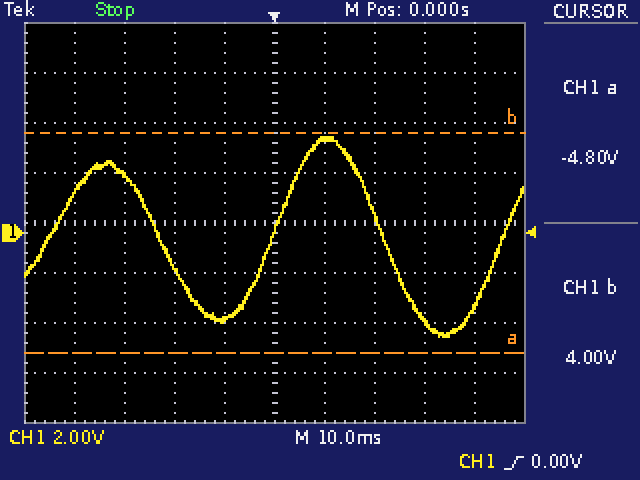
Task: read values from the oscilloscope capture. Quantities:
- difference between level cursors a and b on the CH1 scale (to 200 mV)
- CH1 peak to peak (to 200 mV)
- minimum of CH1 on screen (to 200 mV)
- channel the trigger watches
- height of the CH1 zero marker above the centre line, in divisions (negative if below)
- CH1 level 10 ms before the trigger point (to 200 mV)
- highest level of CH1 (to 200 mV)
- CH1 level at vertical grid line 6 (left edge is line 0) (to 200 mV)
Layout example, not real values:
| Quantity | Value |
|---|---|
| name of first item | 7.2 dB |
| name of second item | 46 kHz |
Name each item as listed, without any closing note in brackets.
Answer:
| Quantity | Value |
|---|---|
| difference between level cursors a and b on the CH1 scale | 8.8 V |
| CH1 peak to peak | 8.0 V |
| minimum of CH1 on screen | -4.2 V |
| channel the trigger watches | CH1 |
| height of the CH1 zero marker above the centre line, in divisions | -0.2 div |
| CH1 level 10 ms before the trigger point | -3.4 V |
| highest level of CH1 | 3.8 V |
| CH1 level at vertical grid line 6 (left edge is line 0) | 3.8 V |
